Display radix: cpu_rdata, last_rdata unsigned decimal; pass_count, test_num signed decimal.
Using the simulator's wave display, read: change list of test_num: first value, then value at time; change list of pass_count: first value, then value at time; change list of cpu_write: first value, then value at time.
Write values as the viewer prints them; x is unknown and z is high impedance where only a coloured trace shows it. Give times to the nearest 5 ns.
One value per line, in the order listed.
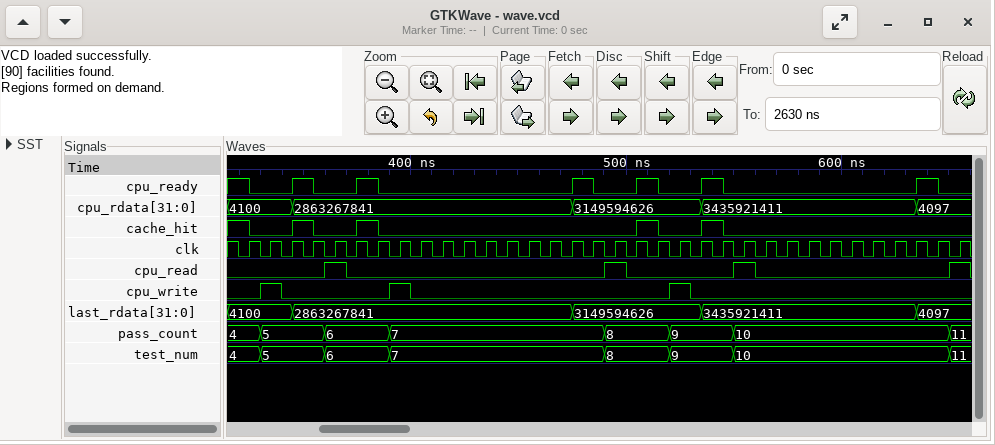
4, 5 at 330 ns, 6 at 360 ns, 7 at 390 ns, 8 at 490 ns, 9 at 520 ns, 10 at 550 ns, 11 at 650 ns
4, 5 at 330 ns, 6 at 360 ns, 7 at 390 ns, 8 at 490 ns, 9 at 520 ns, 10 at 550 ns, 11 at 650 ns
0, 1 at 330 ns, 0 at 340 ns, 1 at 390 ns, 0 at 400 ns, 1 at 520 ns, 0 at 530 ns
